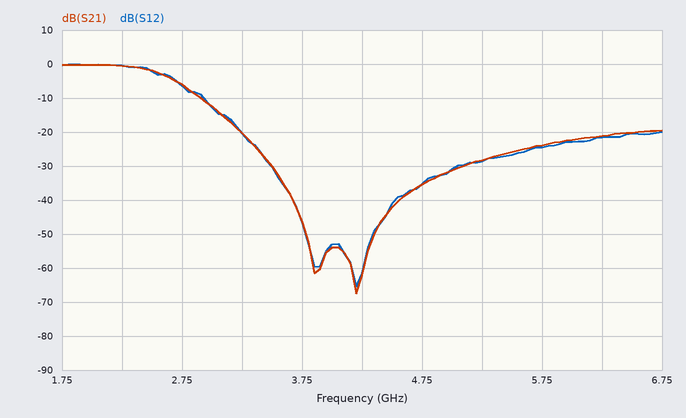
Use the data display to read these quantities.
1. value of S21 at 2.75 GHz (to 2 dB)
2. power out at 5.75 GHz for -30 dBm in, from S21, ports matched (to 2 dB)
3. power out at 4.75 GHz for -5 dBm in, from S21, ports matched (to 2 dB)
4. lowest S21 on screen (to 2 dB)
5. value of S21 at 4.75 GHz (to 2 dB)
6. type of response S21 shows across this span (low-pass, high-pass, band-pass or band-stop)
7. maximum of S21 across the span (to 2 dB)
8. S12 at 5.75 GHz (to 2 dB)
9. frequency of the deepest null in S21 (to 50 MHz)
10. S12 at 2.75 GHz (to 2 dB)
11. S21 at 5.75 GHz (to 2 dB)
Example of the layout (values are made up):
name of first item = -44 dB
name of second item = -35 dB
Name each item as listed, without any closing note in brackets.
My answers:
value of S21 at 2.75 GHz = -6 dB
power out at 5.75 GHz for -30 dBm in, from S21, ports matched = -54 dBm
power out at 4.75 GHz for -5 dBm in, from S21, ports matched = -40 dBm
lowest S21 on screen = -68 dB
value of S21 at 4.75 GHz = -36 dB
type of response S21 shows across this span = low-pass
maximum of S21 across the span = 0 dB
S12 at 5.75 GHz = -24 dB
frequency of the deepest null in S21 = 4.20 GHz
S12 at 2.75 GHz = -6 dB
S21 at 5.75 GHz = -24 dB
